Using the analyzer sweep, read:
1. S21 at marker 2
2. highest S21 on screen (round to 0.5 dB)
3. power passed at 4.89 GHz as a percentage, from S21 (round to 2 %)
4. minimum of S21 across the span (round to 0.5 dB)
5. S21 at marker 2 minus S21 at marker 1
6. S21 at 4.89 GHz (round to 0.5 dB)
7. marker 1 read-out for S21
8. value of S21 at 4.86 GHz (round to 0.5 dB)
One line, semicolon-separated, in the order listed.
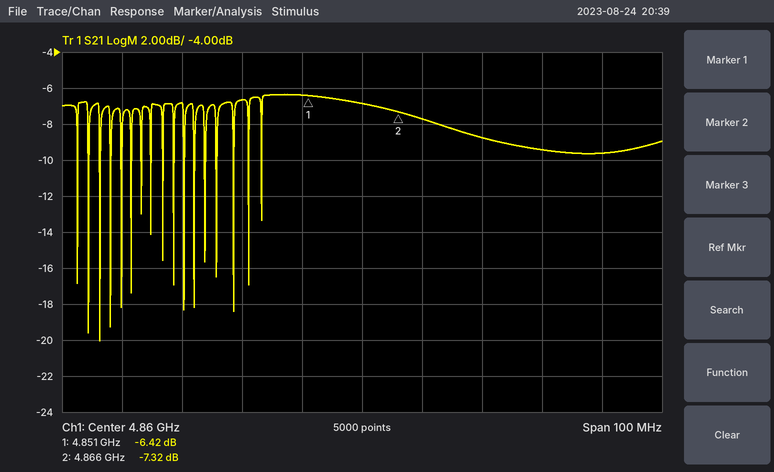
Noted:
-7.32 dB; -6.5 dB; 12 %; -20.0 dB; -0.90 dB; -9.5 dB; -6.42 dB; -7.0 dB
